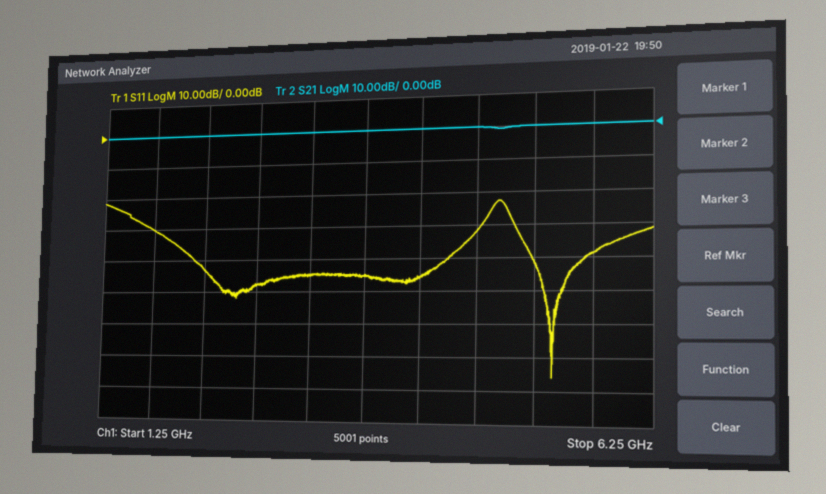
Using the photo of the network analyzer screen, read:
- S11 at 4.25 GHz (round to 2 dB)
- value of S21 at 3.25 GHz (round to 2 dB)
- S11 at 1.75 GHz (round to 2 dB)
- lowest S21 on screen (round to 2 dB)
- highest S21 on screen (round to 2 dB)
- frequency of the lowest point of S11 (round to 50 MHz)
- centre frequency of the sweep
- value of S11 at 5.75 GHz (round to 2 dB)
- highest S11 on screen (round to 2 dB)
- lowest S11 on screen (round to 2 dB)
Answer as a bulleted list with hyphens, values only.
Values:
- -46 dB
- 0 dB
- -30 dB
- 0 dB
- 0 dB
- 5.40 GHz
- 3.75 GHz
- -38 dB
- -22 dB
- -76 dB
